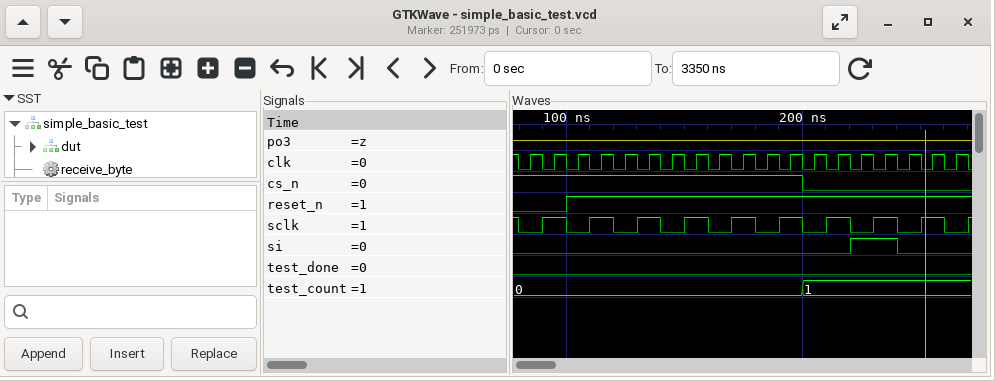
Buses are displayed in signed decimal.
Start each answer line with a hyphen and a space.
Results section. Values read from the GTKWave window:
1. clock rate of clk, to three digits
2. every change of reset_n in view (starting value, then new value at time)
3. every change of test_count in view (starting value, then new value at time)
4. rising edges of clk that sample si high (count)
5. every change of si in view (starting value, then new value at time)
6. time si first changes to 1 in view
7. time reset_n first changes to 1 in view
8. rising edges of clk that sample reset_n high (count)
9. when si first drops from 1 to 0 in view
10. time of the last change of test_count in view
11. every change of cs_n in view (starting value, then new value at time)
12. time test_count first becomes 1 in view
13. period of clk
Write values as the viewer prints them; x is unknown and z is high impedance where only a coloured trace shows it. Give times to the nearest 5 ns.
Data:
- 100 MHz
- 0, 1 at 100 ns
- 0, 1 at 200 ns
- 2
- 0, 1 at 220 ns, 0 at 240 ns
- 220 ns
- 100 ns
- 17
- 240 ns
- 200 ns
- 1, 0 at 200 ns
- 200 ns
- 10 ns
